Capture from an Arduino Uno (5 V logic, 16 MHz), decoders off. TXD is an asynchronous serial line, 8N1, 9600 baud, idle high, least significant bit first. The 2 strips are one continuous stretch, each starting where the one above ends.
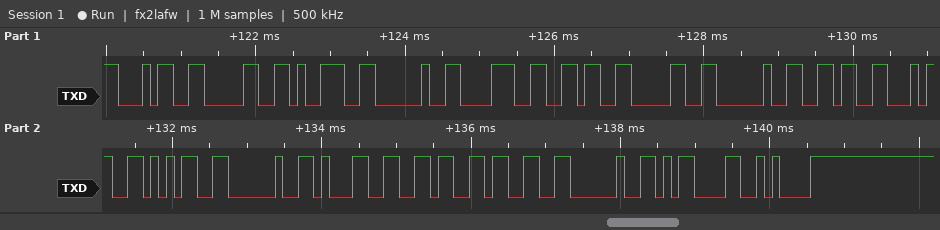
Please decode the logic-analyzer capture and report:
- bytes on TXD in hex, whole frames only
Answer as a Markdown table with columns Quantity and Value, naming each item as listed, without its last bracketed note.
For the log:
| Quantity | Value |
|---|---|
| bytes on TXD in hex, whole frames only | 34 30 39 20 38 36 30 20 36 34 35 20 31 36 33 20 0D 0A |
